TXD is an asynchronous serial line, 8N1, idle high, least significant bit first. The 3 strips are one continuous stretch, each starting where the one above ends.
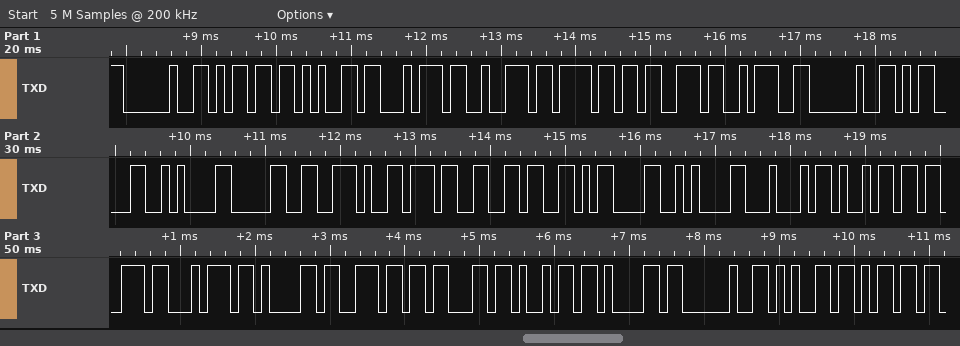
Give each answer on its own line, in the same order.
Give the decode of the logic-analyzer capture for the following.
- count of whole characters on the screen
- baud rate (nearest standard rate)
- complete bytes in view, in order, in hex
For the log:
29
9600 baud
20 6D 65 74 72 6F 73 3A 20 0D 0A 30 2E 37 36 0D 0A 44 69 73 74 61 6E 63 69 61 20 65 6D
